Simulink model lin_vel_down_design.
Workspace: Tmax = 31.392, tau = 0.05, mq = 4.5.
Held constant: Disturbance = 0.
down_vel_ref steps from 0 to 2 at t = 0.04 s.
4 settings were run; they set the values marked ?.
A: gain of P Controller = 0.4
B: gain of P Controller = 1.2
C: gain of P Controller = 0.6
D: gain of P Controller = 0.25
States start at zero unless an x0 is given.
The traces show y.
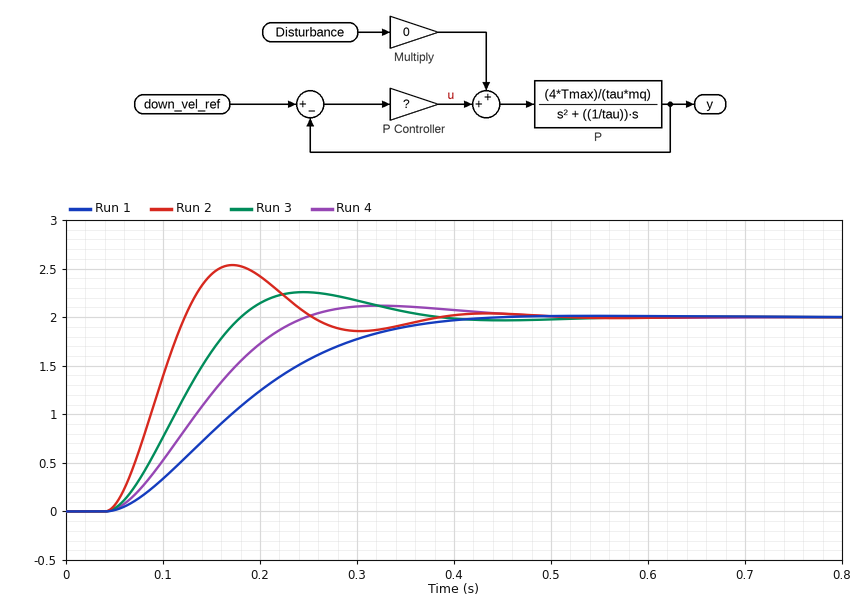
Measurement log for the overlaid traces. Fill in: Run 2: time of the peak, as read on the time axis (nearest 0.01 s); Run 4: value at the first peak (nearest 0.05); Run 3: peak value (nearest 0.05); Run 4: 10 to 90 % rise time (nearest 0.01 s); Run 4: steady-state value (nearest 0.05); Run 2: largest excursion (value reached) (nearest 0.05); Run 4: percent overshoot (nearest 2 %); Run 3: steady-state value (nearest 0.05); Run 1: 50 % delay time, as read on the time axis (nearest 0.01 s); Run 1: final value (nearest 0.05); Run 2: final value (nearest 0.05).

0.17 s
2.10
2.25
0.14 s
2.00
2.55
6 %
2.00
0.17 s
2.00
2.00
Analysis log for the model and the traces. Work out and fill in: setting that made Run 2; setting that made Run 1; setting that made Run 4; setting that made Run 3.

B
D
A
C
